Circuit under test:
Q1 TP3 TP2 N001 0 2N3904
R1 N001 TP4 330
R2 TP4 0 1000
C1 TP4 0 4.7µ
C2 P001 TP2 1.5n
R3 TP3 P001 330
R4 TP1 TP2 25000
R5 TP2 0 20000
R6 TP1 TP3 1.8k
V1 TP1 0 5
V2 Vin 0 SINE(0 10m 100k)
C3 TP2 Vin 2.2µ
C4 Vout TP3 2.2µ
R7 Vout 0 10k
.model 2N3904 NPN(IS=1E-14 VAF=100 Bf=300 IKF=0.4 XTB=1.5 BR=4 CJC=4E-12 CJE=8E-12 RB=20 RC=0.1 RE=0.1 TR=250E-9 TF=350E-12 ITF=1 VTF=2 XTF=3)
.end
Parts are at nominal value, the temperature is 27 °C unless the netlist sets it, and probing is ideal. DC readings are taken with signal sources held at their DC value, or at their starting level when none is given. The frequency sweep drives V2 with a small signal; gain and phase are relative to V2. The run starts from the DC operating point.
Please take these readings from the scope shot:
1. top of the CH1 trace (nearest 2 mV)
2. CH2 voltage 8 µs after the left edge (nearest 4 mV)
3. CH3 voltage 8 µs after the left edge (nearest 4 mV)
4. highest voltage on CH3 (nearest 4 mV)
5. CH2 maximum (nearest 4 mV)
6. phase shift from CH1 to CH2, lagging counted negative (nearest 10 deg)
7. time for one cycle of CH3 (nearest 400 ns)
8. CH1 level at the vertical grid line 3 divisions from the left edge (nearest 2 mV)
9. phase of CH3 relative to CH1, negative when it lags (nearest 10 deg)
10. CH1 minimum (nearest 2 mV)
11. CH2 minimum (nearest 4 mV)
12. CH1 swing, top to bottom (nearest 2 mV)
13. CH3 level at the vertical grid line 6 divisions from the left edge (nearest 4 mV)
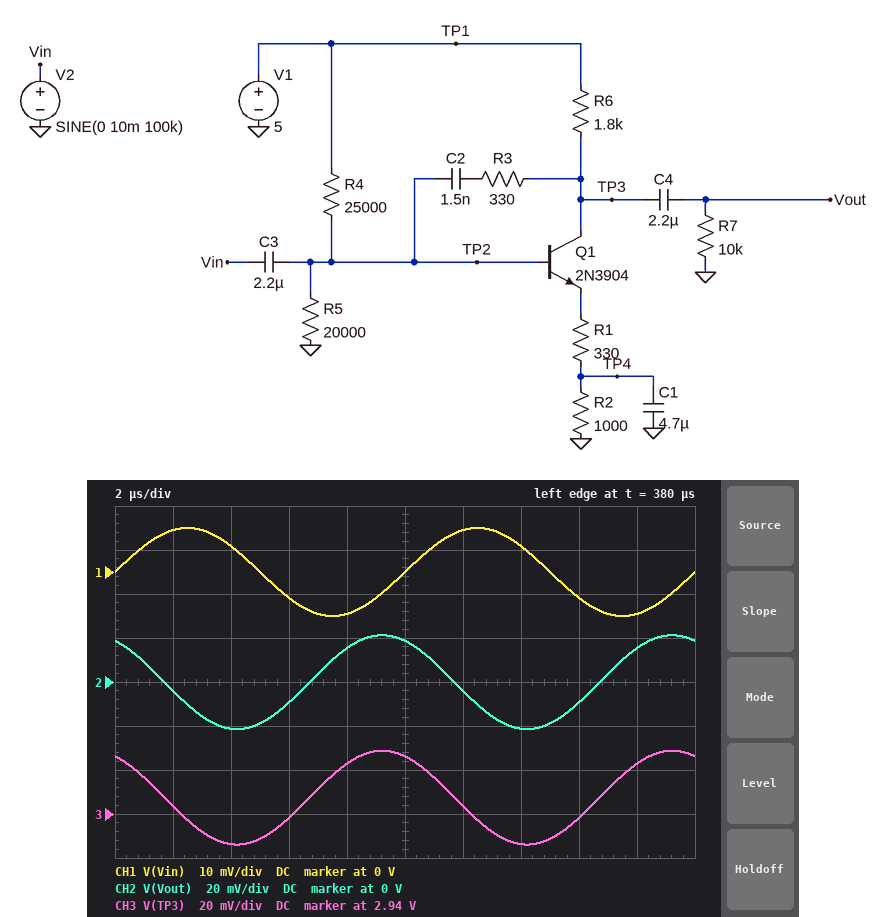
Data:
10 mV
16 mV
2.964 V
2.968 V
20 mV
120 deg
10.0 µs
-6 mV
120 deg
-10 mV
-20 mV
20 mV
2.944 V
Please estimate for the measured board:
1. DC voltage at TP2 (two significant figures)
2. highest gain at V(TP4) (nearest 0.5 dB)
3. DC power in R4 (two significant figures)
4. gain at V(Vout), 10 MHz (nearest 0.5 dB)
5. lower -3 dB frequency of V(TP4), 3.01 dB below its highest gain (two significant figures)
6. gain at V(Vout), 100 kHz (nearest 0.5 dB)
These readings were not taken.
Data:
2.2 V
-3.0 dB
320 µW
-18.0 dB
6.1 Hz
6.5 dB
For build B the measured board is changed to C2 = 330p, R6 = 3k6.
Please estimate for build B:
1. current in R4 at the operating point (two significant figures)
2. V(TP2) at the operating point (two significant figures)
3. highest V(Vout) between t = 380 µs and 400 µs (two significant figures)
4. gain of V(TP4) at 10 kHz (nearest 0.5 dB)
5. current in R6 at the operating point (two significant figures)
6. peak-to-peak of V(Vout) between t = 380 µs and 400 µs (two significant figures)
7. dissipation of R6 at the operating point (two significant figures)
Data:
120 µA
2.0 V
25 mV
-42.0 dB
990 µA
36 mV
3.6 mW
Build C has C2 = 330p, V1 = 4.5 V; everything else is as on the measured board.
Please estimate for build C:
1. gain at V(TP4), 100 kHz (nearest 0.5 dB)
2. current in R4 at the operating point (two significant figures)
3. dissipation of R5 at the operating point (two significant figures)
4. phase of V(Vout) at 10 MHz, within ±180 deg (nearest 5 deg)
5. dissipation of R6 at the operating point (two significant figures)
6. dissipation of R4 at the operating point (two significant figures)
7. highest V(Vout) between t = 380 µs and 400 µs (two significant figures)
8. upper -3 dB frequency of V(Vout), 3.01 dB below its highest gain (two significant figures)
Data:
-60.5 dB
100 µA
190 µW
65 deg
1.7 mW
260 µW
40 mV
260 kHz
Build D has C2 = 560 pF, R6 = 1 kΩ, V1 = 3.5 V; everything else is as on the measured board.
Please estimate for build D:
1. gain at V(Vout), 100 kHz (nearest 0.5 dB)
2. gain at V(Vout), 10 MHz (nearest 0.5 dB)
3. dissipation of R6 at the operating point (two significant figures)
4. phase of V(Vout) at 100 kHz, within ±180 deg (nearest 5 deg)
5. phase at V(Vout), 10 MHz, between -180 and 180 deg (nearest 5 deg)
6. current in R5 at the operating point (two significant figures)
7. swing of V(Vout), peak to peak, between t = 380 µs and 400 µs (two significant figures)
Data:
7.0 dB
-16.0 dB
440 µW
155 deg
55 deg
77 µA
45 mV
